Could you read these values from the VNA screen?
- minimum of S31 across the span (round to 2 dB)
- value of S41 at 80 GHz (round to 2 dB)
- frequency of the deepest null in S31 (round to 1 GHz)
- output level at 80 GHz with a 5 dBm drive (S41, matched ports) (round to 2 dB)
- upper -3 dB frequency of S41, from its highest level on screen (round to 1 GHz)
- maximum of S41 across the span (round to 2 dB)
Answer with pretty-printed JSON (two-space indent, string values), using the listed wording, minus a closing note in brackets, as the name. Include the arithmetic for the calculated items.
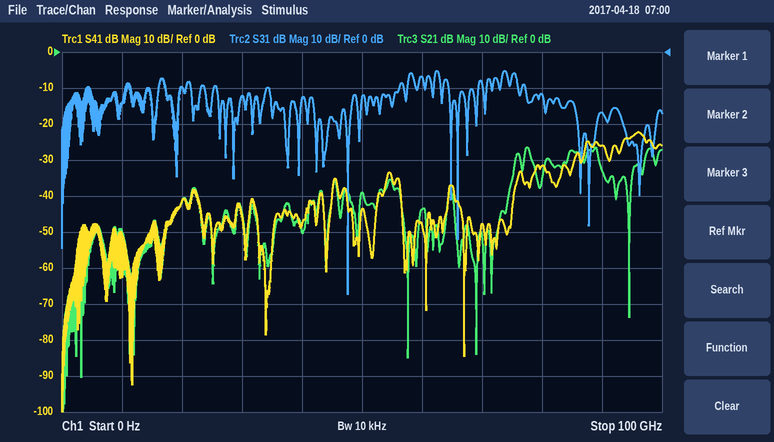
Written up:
{
  "minimum of S31 across the span": "-68 dB",
  "value of S41 at 80 GHz": "-32 dB",
  "frequency of the deepest null in S31": "48 GHz",
  "output level at 80 GHz with a 5 dBm drive (S41, matched ports)": "5 dBm + (-32 dB) = -26 dBm",
  "upper -3 dB frequency of S41, from its highest level on screen": "98 GHz",
  "maximum of S41 across the span": "-22 dB"
}
